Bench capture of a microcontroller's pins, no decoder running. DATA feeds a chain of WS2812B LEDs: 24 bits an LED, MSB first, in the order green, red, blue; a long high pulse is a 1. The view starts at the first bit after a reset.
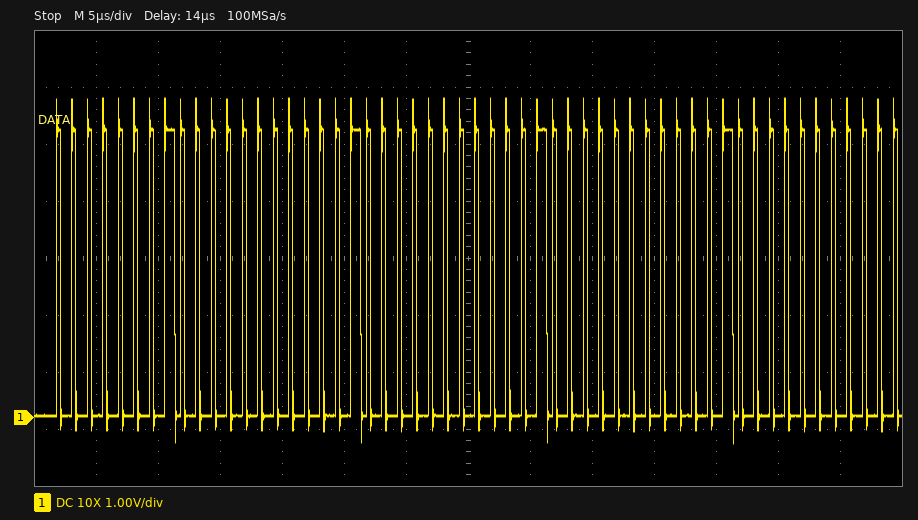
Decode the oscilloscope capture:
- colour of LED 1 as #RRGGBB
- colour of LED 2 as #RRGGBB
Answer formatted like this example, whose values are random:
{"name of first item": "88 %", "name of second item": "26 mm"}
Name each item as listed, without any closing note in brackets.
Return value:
{"colour of LED 1 as #RRGGBB": "#000110", "colour of LED 2 as #RRGGBB": "#000110"}
